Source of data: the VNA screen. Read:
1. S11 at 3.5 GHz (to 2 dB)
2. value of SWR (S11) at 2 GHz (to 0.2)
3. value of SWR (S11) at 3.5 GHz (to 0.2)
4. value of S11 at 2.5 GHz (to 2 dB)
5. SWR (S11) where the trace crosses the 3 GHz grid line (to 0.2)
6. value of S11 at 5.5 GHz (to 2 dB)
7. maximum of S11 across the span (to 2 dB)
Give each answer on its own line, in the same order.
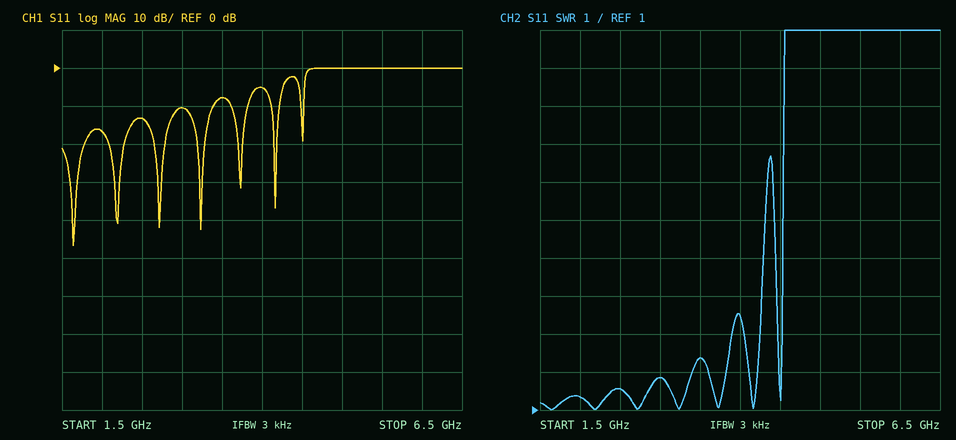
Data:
-8 dB
1.4
2.4
-14 dB
1.8
0 dB
0 dB
